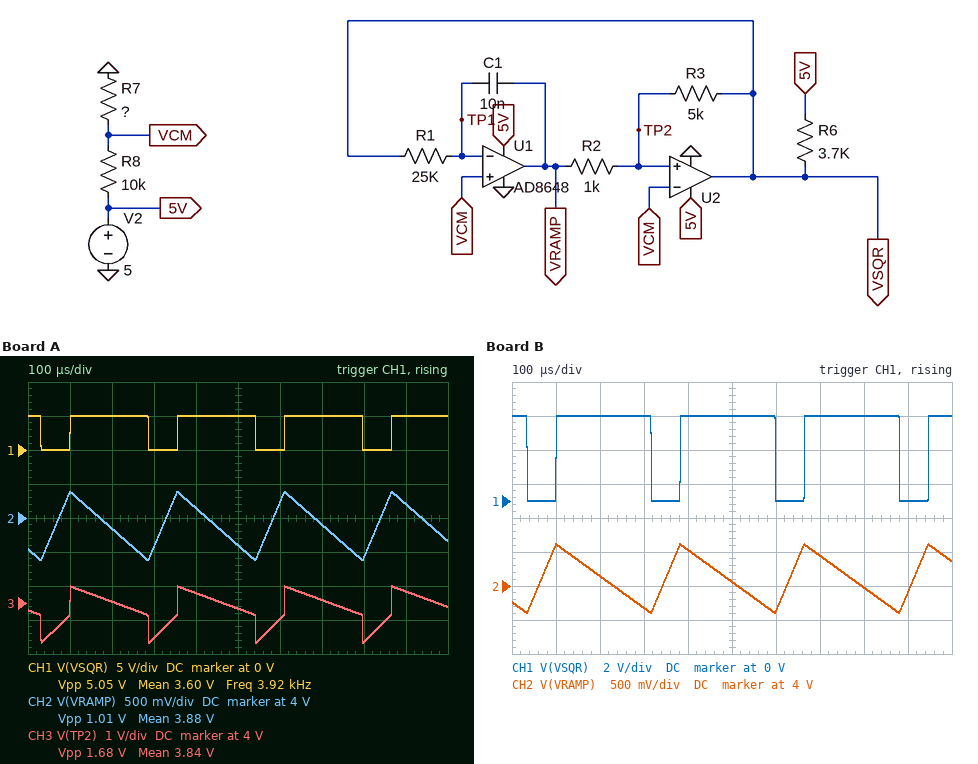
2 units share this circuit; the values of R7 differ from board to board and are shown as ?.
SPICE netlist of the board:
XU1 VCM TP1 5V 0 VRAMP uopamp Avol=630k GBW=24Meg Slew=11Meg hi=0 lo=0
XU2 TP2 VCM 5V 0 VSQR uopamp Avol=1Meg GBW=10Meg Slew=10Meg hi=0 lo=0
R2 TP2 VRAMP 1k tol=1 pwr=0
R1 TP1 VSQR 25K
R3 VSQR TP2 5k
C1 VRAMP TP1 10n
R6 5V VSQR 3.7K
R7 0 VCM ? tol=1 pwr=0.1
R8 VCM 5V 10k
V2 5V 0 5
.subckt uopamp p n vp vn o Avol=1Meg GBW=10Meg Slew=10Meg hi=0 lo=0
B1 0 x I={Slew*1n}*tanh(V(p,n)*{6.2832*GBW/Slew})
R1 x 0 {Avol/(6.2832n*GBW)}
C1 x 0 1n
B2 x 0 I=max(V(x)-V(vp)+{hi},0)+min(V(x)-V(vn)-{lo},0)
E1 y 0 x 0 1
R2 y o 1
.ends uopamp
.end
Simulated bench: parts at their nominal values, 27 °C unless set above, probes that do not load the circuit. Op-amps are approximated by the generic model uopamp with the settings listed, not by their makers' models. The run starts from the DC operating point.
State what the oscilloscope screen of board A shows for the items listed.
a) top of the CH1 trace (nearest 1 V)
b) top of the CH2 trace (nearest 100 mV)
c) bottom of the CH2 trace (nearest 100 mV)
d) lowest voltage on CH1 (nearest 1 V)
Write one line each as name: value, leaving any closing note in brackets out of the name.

top of the CH1 trace: 5 V
top of the CH2 trace: 4.4 V
bottom of the CH2 trace: 3.4 V
lowest voltage on CH1: 0 V
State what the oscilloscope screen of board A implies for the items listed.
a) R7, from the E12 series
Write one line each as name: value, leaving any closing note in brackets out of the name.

R7, from the E12 series: 27 kΩ
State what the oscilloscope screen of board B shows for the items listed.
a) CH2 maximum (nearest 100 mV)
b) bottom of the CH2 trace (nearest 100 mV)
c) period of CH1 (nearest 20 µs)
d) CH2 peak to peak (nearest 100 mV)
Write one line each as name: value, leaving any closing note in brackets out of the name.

CH2 maximum: 4.6 V
bottom of the CH2 trace: 3.6 V
period of CH1: 280 µs
CH2 peak to peak: 1.0 V
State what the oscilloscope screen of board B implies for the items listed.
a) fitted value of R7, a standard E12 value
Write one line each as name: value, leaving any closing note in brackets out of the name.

fitted value of R7, a standard E12 value: 33 kΩ
